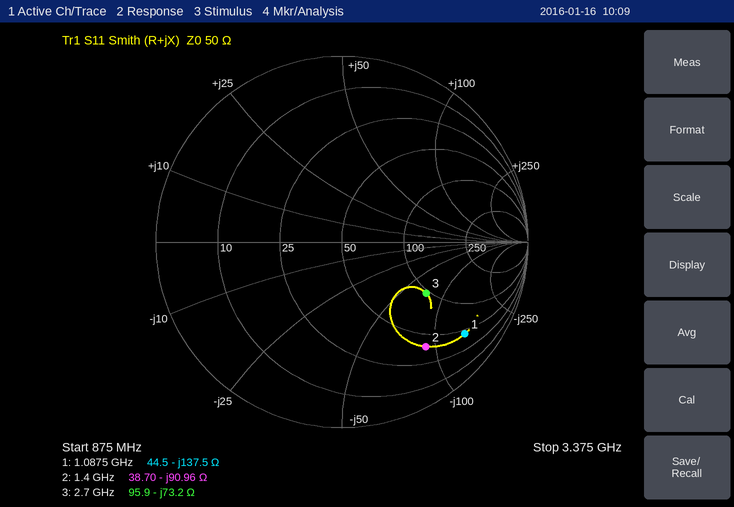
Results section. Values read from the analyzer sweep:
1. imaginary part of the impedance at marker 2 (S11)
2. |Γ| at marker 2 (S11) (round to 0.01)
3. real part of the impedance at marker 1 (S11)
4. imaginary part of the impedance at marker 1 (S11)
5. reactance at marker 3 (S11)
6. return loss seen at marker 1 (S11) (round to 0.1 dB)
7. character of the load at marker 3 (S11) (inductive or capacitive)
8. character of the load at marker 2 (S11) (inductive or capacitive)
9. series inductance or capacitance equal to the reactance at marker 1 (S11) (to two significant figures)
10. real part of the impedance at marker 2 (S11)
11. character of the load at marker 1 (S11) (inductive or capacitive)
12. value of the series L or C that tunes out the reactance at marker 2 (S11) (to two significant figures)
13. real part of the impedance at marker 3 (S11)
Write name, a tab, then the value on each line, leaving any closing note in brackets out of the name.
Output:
imaginary part of the impedance at marker 2	-90.96 Ω
|Γ| at marker 2 (S11)	0.72
real part of the impedance at marker 1	44.5 Ω
imaginary part of the impedance at marker 1	-137.5 Ω
reactance at marker 3	-73.2 Ω
return loss seen at marker 1 (S11)	1.7 dB
character of the load at marker 3 (S11)	capacitive
character of the load at marker 2 (S11)	capacitive
series inductance or capacitance equal to the reactance at marker 1 (S11)	1.1 pF
real part of the impedance at marker 2	38.70 Ω
character of the load at marker 1 (S11)	capacitive
value of the series L or C that tunes out the reactance at marker 2 (S11)	10 nH
real part of the impedance at marker 3	95.9 Ω
